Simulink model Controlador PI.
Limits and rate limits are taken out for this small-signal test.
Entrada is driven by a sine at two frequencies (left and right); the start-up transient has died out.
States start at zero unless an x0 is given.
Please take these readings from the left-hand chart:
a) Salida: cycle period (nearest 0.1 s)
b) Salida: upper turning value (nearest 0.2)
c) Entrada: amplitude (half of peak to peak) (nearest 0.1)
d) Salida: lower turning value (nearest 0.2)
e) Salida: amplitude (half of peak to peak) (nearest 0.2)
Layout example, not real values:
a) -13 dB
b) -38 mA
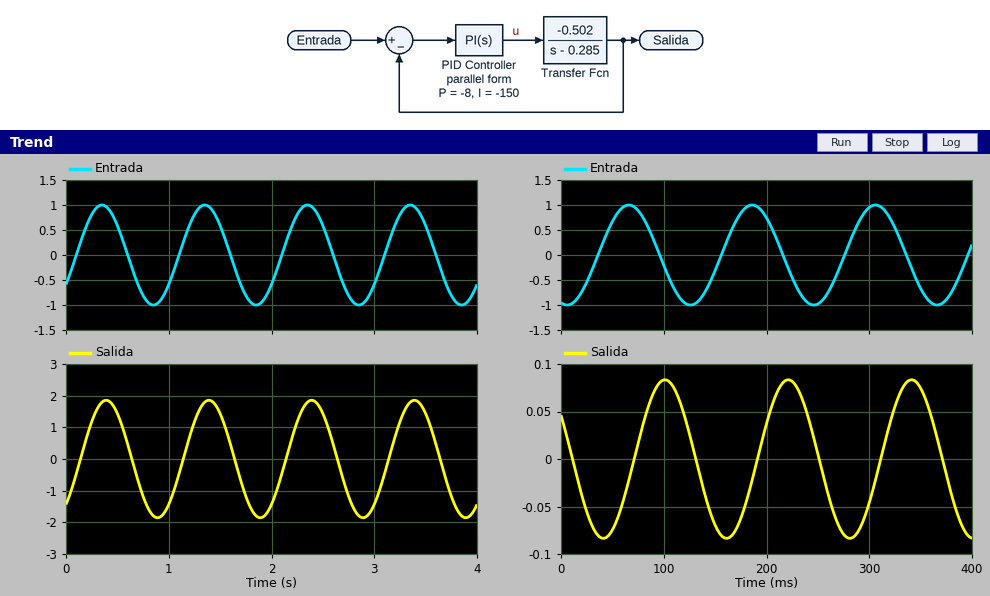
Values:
a) 1.0 s
b) 1.8
c) 1.0
d) -1.8
e) 1.8
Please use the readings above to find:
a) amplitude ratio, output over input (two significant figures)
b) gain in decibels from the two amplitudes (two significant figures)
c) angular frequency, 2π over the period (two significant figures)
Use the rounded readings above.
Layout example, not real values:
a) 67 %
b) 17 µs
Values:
a) 1.8
b) 5.1 dB
c) 6.3 rad/s
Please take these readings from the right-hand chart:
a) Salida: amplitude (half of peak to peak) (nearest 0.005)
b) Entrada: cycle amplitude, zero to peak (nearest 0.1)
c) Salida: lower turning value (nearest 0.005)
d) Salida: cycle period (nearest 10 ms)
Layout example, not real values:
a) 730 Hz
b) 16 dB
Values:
a) 0.085
b) 1.0
c) -0.085
d) 120 ms
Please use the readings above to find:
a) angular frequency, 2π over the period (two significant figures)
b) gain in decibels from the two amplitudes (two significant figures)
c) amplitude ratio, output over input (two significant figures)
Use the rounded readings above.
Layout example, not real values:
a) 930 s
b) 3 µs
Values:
a) 0.052 rad/ms
b) -21 dB
c) 0.085
